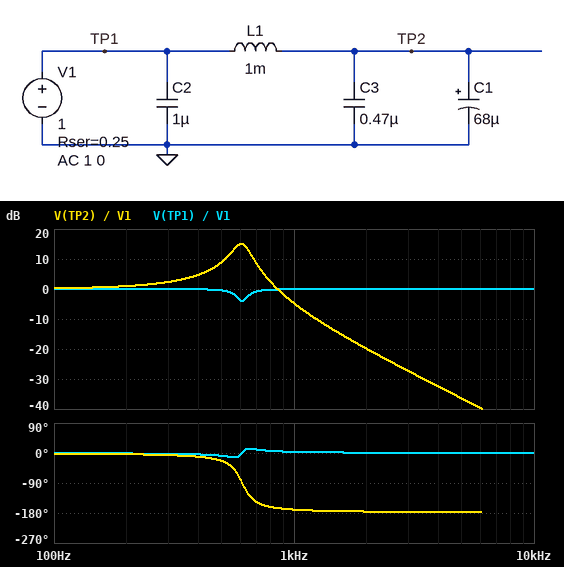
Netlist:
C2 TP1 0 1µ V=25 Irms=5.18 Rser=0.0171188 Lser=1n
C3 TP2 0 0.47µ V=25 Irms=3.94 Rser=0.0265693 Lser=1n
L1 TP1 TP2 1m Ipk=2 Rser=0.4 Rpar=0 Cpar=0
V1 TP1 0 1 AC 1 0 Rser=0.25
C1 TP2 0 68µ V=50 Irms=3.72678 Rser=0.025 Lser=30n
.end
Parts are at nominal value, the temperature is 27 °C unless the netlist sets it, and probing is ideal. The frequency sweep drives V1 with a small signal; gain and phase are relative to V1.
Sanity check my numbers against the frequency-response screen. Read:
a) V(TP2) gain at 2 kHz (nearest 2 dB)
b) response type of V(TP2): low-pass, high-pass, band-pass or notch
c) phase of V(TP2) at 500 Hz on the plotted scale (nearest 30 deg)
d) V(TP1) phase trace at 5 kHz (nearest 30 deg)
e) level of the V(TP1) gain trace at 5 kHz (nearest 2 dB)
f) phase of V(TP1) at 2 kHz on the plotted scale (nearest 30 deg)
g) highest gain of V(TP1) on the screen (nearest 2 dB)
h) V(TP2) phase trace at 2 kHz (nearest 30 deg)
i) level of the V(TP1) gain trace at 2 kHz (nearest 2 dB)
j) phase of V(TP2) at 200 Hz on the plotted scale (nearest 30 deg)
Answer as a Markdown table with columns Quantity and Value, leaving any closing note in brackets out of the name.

| Quantity | Value |
|---|---|
| V(TP2) gain at 2 kHz | -20 dB |
| response type of V(TP2): low-pass, high-pass, band-pass or notch | band-pass |
| phase of V(TP2) at 500 Hz on the plotted scale | -30 deg |
| V(TP1) phase trace at 5 kHz | 0 deg |
| level of the V(TP1) gain trace at 5 kHz | 0 dB |
| phase of V(TP1) at 2 kHz on the plotted scale | 0 deg |
| highest gain of V(TP1) on the screen | 0 dB |
| V(TP2) phase trace at 2 kHz | -180 deg |
| level of the V(TP1) gain trace at 2 kHz | 0 dB |
| phase of V(TP2) at 200 Hz on the plotted scale | 0 deg |
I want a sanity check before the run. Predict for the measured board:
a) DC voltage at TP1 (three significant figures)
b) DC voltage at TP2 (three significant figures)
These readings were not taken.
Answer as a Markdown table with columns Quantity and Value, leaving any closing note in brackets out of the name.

| Quantity | Value |
|---|---|
| DC voltage at TP1 | 1.00 V |
| DC voltage at TP2 | 1.00 V |
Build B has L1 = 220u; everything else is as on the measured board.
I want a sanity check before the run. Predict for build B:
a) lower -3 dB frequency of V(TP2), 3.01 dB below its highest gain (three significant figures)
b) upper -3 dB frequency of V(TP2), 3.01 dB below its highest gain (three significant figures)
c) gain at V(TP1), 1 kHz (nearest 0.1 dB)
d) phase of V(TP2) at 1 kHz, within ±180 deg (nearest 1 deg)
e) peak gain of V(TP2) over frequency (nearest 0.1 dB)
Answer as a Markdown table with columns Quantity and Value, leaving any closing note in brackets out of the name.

| Quantity | Value |
|---|---|
| lower -3 dB frequency of V(TP2), 3.01 dB below its highest gain | 970 Hz |
| upper -3 dB frequency of V(TP2), 3.01 dB below its highest gain | 1.48 kHz |
| gain at V(TP1), 1 kHz | -1.0 dB |
| phase of V(TP2) at 1 kHz, within ±180 deg | -35 deg |
| peak gain of V(TP2) over frequency | 8.6 dB |
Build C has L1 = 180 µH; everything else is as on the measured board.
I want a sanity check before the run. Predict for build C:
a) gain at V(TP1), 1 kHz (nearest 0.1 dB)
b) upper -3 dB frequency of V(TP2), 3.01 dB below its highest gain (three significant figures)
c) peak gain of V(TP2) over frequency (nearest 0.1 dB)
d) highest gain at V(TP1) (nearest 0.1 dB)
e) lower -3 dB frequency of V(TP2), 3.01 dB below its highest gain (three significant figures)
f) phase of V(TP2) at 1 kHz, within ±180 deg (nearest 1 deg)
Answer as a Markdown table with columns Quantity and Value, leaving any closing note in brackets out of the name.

| Quantity | Value |
|---|---|
| gain at V(TP1), 1 kHz | -0.7 dB |
| upper -3 dB frequency of V(TP2), 3.01 dB below its highest gain | 1.65 kHz |
| peak gain of V(TP2) over frequency | 7.8 dB |
| highest gain at V(TP1) | 0 dB |
| lower -3 dB frequency of V(TP2), 3.01 dB below its highest gain | 1.02 kHz |
| phase of V(TP2) at 1 kHz, within ±180 deg | -29 deg |
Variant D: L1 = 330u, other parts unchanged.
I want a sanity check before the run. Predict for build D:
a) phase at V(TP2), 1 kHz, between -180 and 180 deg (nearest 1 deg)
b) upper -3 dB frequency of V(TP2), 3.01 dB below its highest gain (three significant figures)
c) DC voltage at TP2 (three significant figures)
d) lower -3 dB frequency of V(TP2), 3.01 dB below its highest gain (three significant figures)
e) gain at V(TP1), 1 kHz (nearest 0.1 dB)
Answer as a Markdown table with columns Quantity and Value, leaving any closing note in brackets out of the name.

| Quantity | Value |
|---|---|
| phase at V(TP2), 1 kHz, between -180 and 180 deg | -69 deg |
| upper -3 dB frequency of V(TP2), 3.01 dB below its highest gain | 1.19 kHz |
| DC voltage at TP2 | 1.00 V |
| lower -3 dB frequency of V(TP2), 3.01 dB below its highest gain | 853 Hz |
| gain at V(TP1), 1 kHz | -3.3 dB |
